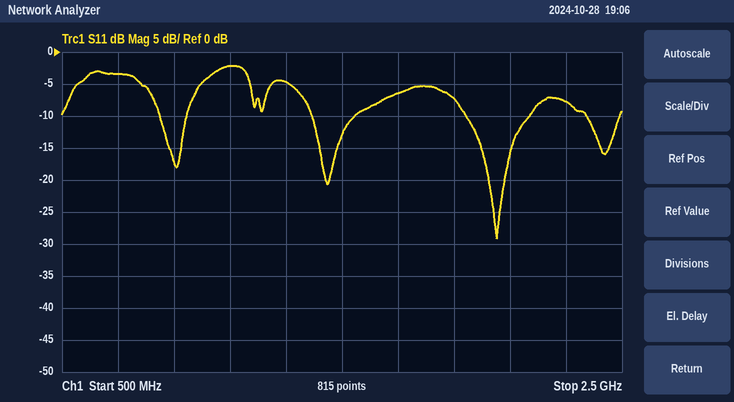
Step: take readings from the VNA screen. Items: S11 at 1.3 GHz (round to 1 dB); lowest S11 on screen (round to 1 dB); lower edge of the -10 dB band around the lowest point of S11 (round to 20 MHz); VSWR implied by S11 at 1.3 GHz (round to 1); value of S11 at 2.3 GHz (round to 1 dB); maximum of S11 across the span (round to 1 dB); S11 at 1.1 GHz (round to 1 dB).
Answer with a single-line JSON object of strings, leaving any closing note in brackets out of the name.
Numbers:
{"S11 at 1.3 GHz": "-5 dB", "lowest S11 on screen": "-29 dB", "lower edge of the -10 dB band around the lowest point of S11": "1.94 GHz", "VSWR implied by S11 at 1.3 GHz": "4", "value of S11 at 2.3 GHz": "-8 dB", "maximum of S11 across the span": "-2 dB", "S11 at 1.1 GHz": "-2 dB"}
